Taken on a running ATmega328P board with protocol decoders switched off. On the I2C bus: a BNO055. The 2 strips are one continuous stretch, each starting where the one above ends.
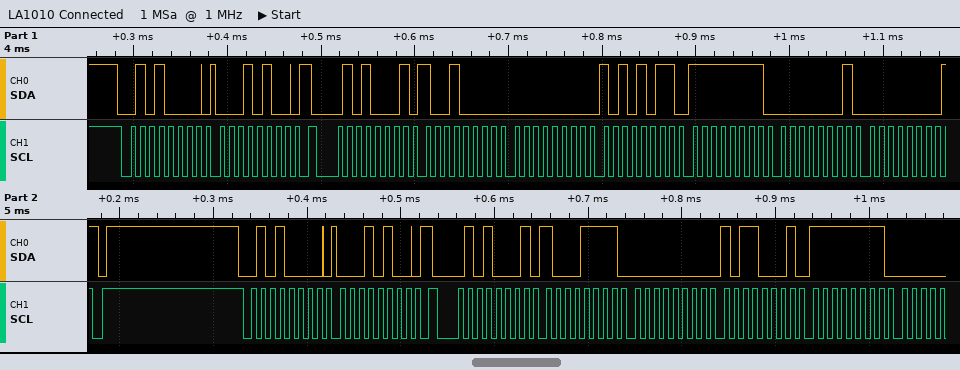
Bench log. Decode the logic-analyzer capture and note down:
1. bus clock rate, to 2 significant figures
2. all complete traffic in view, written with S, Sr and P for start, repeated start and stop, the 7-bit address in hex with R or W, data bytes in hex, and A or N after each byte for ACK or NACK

100 kHz
S 28W A 14 A Sr 28R A 90 A 00 A AB A FF A 01 A 00 N P S 28W A 14 A Sr 28R A 8F A 00 A B1 A FF A
